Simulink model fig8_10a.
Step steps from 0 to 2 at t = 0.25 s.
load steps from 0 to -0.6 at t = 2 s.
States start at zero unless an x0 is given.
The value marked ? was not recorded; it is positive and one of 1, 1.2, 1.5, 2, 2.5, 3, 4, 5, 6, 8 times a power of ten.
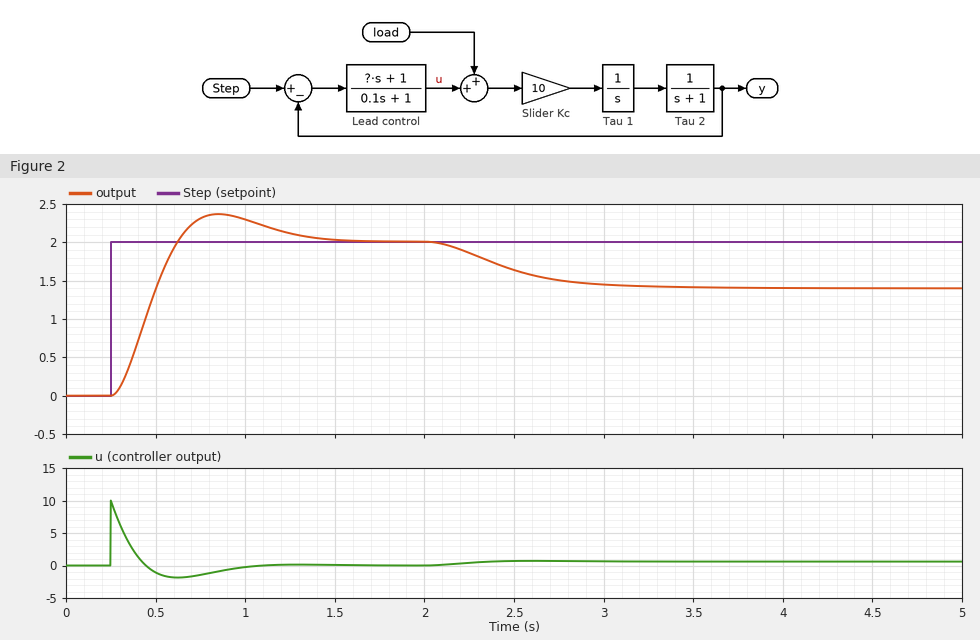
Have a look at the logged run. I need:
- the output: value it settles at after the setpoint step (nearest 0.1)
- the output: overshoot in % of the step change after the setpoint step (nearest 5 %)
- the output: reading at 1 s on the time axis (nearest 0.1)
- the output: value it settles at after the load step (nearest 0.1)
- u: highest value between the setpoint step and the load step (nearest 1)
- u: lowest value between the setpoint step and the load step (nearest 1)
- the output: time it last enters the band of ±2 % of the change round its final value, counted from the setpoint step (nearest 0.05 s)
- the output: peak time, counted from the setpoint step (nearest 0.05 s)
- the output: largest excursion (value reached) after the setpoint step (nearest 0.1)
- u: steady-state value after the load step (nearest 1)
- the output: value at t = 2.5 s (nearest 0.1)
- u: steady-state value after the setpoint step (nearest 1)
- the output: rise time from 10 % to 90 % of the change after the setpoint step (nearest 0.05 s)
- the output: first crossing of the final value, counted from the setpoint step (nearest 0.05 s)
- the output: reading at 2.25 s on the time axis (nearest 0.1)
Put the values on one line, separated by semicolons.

2.0; 20 %; 2.3; 1.4; 10; -2; 1.20 s; 0.60 s; 2.4; 1; 1.6; 0; 0.25 s; 0.35 s; 1.9
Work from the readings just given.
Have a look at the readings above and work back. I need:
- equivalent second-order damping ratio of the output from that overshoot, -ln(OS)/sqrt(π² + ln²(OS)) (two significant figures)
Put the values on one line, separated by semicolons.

0.46
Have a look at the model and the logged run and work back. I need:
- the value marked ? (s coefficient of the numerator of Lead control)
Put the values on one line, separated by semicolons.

0.5
